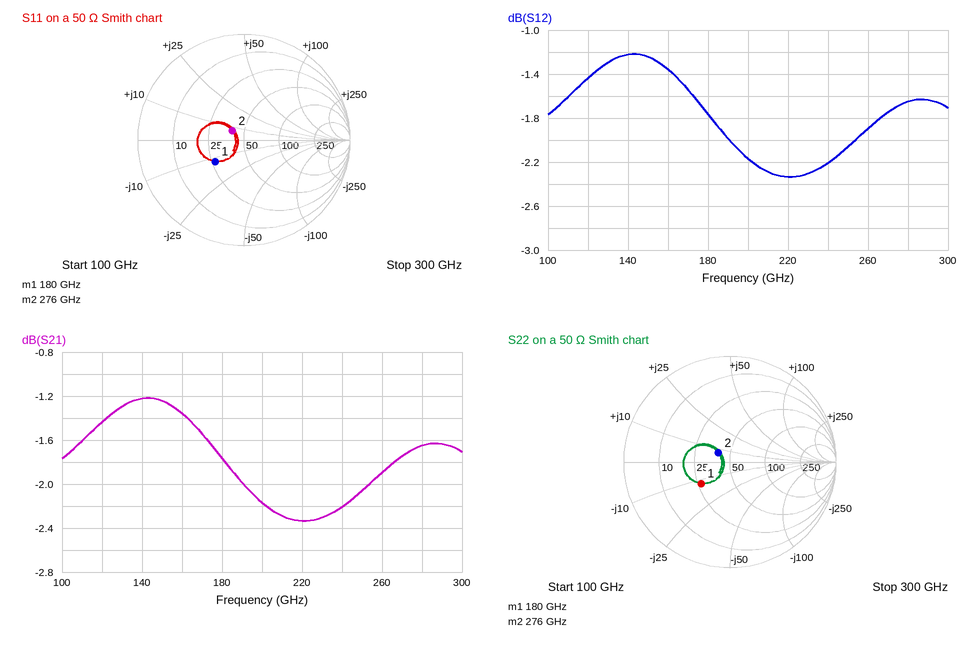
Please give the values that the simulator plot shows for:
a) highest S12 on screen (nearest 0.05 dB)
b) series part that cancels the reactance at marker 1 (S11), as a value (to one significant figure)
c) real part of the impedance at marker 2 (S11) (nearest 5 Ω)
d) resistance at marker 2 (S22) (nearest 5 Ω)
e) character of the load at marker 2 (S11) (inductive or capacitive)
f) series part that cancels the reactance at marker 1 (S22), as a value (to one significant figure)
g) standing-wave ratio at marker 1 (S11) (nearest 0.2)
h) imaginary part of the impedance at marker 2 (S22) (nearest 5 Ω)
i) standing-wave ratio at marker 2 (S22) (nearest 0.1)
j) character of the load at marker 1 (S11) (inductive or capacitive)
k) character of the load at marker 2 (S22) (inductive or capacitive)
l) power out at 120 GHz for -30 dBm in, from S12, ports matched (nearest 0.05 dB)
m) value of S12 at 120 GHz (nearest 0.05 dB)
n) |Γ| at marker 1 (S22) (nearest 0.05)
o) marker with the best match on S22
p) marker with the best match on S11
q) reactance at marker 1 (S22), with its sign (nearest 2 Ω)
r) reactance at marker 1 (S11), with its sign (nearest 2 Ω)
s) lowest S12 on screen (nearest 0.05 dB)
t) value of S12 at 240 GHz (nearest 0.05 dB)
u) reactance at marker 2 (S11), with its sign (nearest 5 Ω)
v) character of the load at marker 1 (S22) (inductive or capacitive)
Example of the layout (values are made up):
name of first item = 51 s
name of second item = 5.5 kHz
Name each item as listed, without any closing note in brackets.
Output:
highest S12 on screen = -1.20 dB
series part that cancels the reactance at marker 1 (S11), as a value = 10 pH
real part of the impedance at marker 2 (S11) = 40 Ω
resistance at marker 2 (S22) = 40 Ω
character of the load at marker 2 (S11) = inductive
series part that cancels the reactance at marker 1 (S22), as a value = 10 pH
standing-wave ratio at marker 1 (S11) = 2.0
imaginary part of the impedance at marker 2 (S22) = +5 Ω
standing-wave ratio at marker 2 (S22) = 1.3
character of the load at marker 1 (S11) = capacitive
character of the load at marker 2 (S22) = inductive
power out at 120 GHz for -30 dBm in, from S12, ports matched = -31.45 dBm
value of S12 at 120 GHz = -1.45 dB
|Γ| at marker 1 (S22) = 0.35
marker with the best match on S22 = marker 2
marker with the best match on S11 = marker 2
reactance at marker 1 (S22), with its sign = -12 Ω
reactance at marker 1 (S11), with its sign = -12 Ω
lowest S12 on screen = -2.35 dB
value of S12 at 240 GHz = -2.20 dB
reactance at marker 2 (S11), with its sign = +5 Ω
character of the load at marker 1 (S22) = capacitive
